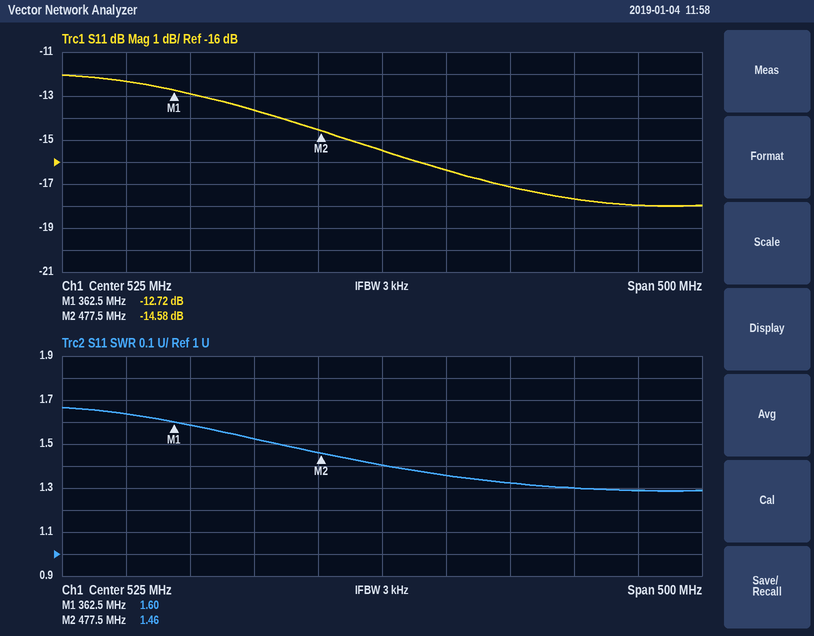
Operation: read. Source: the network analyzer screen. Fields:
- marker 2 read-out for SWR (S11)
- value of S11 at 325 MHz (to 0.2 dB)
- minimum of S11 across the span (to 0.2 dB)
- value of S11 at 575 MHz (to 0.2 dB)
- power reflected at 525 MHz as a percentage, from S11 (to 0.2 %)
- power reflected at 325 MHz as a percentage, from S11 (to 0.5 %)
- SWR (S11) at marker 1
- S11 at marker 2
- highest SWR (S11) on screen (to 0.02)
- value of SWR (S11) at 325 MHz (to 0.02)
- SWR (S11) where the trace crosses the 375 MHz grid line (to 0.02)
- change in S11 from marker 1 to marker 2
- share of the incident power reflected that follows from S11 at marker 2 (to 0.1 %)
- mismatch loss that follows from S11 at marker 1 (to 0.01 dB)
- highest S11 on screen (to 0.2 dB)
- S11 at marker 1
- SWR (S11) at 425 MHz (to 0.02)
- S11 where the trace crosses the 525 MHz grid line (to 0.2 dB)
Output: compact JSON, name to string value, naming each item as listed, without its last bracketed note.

{"marker 2 read-out for SWR": "1.46", "value of S11 at 325 MHz": "-12.4 dB", "minimum of S11 across the span": "-18.0 dB", "value of S11 at 575 MHz": "-16.4 dB", "power reflected at 525 MHz as a percentage, from S11": "2.8 %", "power reflected at 325 MHz as a percentage, from S11": "6.0 %", "SWR (S11) at marker 1": "1.60", "S11 at marker 2": "-14.58 dB", "highest SWR (S11) on screen": "1.66", "value of SWR (S11) at 325 MHz": "1.64", "SWR (S11) where the trace crosses the 375 MHz grid line": "1.58", "change in S11 from marker 1 to marker 2": "-1.86 dB", "share of the incident power reflected that follows from S11 at marker 2": "3.5 %", "mismatch loss that follows from S11 at marker 1": "0.24 dB", "highest S11 on screen": "-12.0 dB", "S11 at marker 1": "-12.72 dB", "SWR (S11) at 425 MHz": "1.52", "S11 where the trace crosses the 525 MHz grid line": "-15.4 dB"}
